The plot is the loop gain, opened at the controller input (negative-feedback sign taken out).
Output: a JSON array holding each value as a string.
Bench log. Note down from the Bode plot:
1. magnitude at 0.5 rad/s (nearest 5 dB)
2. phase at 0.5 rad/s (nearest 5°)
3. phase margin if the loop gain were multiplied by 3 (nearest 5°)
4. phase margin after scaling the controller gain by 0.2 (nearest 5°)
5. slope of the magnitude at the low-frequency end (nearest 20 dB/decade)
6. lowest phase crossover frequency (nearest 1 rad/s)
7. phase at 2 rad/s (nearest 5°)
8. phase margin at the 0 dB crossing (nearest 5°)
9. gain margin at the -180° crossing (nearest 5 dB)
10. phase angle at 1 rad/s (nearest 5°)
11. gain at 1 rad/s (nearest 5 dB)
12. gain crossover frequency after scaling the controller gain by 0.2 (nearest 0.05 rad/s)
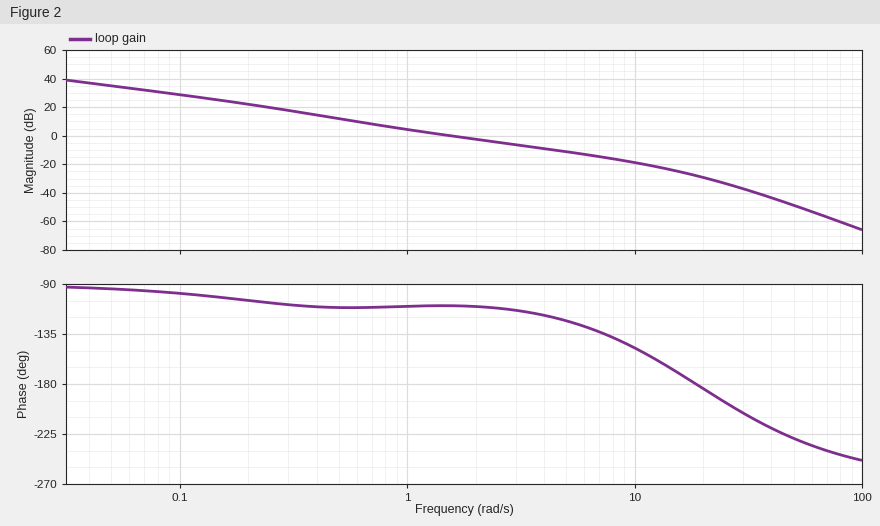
["10 dB", "-110°", "60°", "70°", "-20 dB/decade", "19 rad/s", "-110°", "70°", "30 dB", "-110°", "5 dB", "0.40 rad/s"]
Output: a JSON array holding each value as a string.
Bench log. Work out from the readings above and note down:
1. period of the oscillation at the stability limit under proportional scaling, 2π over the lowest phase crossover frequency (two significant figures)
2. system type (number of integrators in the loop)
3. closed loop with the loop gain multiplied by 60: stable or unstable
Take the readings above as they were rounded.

["0.33 s", "1", "unstable"]
